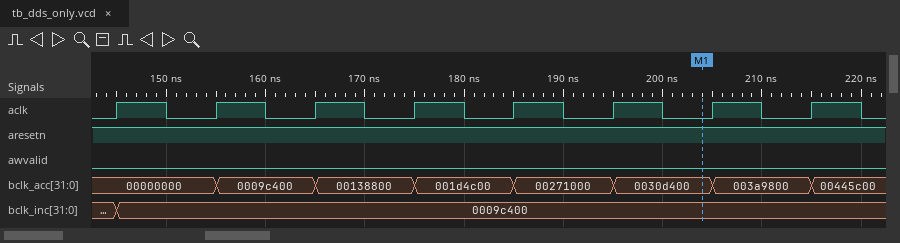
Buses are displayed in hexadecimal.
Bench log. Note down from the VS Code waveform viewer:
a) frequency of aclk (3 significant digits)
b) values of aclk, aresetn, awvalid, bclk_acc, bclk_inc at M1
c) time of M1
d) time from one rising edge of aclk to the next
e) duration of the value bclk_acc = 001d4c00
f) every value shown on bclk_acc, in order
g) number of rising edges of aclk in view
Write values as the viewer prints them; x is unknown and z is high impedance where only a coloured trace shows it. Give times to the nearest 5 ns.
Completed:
100 MHz
aclk=0, aresetn=1, awvalid=0, bclk_acc=0030d400, bclk_inc=0009c400
205 ns
10 ns
10 ns
00000000, 0009c400, 00138800, 001d4c00, 00271000, 0030d400, 003a9800, 00445c00
8
